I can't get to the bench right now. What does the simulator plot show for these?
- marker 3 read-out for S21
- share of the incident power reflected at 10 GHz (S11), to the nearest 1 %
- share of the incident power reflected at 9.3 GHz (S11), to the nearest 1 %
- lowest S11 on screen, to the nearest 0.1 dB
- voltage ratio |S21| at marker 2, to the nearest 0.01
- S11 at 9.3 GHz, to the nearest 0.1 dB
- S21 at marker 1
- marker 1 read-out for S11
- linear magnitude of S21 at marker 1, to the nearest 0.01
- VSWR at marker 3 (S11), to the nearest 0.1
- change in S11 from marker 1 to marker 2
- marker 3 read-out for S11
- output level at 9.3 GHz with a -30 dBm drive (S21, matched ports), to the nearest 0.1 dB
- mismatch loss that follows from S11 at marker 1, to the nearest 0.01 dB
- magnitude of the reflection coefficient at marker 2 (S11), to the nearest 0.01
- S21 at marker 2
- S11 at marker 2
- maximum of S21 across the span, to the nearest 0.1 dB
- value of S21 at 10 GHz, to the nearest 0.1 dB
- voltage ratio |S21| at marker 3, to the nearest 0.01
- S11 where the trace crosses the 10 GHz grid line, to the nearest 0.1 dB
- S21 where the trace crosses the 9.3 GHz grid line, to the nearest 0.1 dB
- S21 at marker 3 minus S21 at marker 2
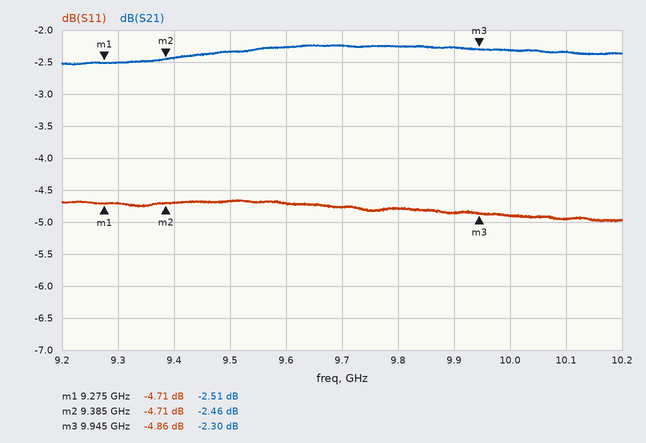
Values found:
-2.30 dB
32 %
34 %
-5.0 dB
0.75
-4.7 dB
-2.51 dB
-4.71 dB
0.75
3.7
0.00 dB
-4.86 dB
-32.5 dBm
1.79 dB
0.58
-2.46 dB
-4.71 dB
-2.2 dB
-2.3 dB
0.77
-4.9 dB
-2.5 dB
0.16 dB
